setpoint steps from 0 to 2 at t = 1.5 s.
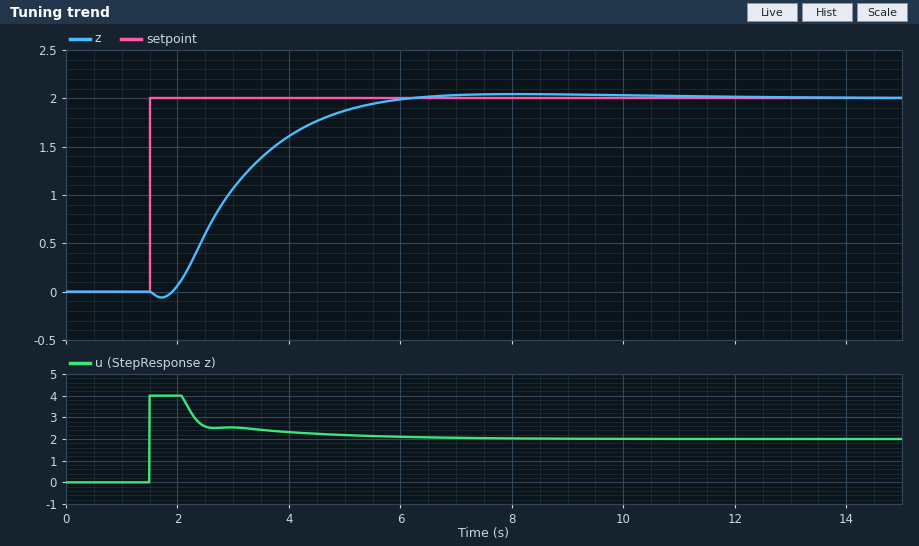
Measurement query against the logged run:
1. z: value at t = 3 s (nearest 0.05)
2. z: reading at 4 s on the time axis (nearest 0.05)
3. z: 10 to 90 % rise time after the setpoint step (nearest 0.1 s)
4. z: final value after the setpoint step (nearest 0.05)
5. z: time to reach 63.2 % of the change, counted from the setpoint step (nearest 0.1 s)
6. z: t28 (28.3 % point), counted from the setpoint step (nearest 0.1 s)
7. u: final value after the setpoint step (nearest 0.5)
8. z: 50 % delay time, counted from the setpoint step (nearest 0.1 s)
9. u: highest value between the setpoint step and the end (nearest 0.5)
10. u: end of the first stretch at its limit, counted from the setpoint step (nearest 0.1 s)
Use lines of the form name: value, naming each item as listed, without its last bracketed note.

z: value at t = 3 s: 1.05
z: reading at 4 s on the time axis: 1.60
z: 10 to 90 % rise time after the setpoint step: 2.5 s
z: final value after the setpoint step: 2.00
z: time to reach 63.2 % of the change, counted from the setpoint step: 1.8 s
z: t28 (28.3 % point), counted from the setpoint step: 1.0 s
u: final value after the setpoint step: 2.0
z: 50 % delay time, counted from the setpoint step: 1.4 s
u: highest value between the setpoint step and the end: 4.0
u: end of the first stretch at its limit, counted from the setpoint step: 0.6 s
